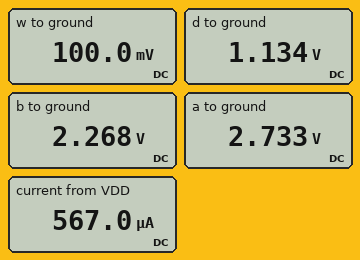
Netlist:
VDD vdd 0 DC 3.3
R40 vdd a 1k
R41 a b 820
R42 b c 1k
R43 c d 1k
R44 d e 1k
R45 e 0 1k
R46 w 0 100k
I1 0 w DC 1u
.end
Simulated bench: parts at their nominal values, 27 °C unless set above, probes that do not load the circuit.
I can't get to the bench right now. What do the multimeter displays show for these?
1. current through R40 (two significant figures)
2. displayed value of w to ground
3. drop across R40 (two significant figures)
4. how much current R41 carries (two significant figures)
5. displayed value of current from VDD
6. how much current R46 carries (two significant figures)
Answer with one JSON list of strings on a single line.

["570 µA", "100.0 mV", "570 mV", "570 µA", "567.0 µA", "1.0 µA"]
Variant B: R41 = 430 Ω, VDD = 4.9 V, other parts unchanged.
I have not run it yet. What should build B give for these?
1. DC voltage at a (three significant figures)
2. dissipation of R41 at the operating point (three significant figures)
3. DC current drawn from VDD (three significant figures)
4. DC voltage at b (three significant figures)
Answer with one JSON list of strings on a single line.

["4.00 V", "350 µW", "902 µA", "3.61 V"]
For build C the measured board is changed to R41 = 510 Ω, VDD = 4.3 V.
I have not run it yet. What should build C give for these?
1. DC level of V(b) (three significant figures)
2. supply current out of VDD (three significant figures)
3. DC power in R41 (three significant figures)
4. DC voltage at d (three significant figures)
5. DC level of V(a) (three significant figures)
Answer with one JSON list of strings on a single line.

["3.12 V", "780 µA", "311 µW", "1.56 V", "3.52 V"]
